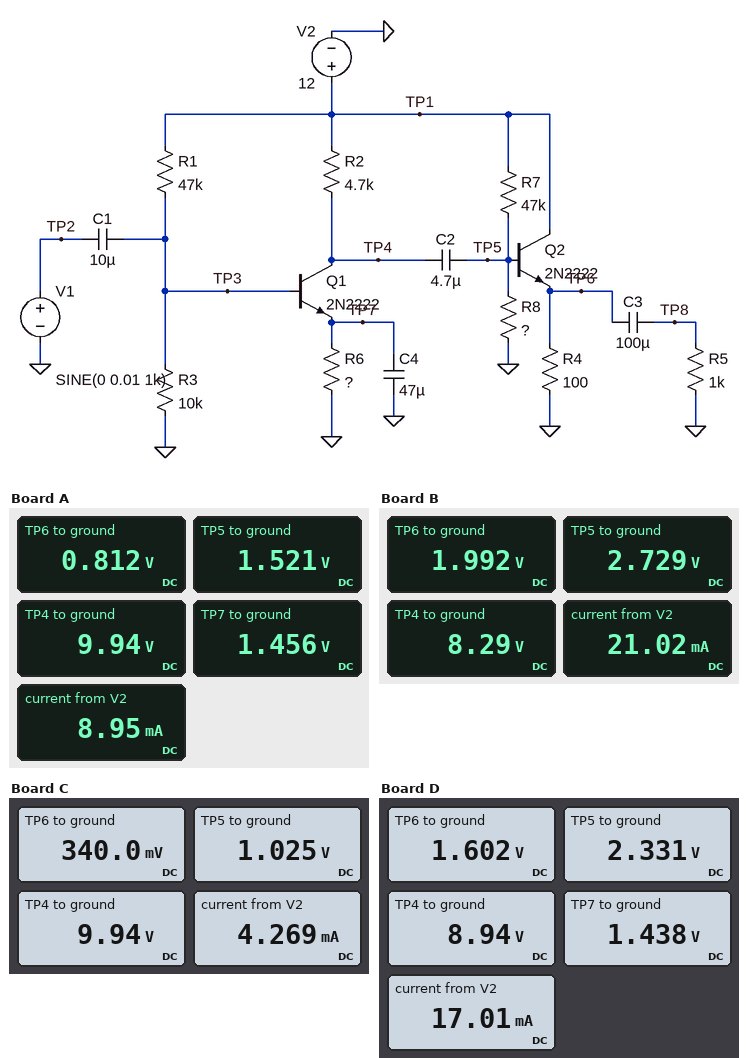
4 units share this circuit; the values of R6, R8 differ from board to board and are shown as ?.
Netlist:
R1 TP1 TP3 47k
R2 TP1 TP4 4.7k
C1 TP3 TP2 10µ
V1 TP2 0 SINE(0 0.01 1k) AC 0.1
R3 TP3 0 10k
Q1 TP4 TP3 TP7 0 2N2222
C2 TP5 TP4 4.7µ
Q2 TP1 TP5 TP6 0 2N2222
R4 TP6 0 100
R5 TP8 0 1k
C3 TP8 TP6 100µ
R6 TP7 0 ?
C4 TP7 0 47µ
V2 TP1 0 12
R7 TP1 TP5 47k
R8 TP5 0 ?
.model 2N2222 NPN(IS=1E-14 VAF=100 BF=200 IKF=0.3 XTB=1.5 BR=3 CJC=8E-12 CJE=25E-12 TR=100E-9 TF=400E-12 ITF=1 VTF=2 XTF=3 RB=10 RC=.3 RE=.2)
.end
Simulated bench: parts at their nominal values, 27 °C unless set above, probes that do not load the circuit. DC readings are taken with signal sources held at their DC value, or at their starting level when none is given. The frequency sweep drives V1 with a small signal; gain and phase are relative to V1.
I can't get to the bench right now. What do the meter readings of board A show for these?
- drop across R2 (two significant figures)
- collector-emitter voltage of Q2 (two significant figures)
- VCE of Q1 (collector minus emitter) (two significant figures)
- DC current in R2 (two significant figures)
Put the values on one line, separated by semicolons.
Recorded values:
2.1 V; 11 V; 8.5 V; 440 µA
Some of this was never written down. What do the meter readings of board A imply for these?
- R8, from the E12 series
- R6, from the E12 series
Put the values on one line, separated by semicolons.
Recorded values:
8.2 kΩ; 3.3 kΩ
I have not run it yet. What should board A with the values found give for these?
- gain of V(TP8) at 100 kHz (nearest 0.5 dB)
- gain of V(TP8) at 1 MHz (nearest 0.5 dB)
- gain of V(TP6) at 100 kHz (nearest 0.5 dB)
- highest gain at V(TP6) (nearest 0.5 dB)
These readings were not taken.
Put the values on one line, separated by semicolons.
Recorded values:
32.0 dB; 32.0 dB; 32.0 dB; 32.0 dB
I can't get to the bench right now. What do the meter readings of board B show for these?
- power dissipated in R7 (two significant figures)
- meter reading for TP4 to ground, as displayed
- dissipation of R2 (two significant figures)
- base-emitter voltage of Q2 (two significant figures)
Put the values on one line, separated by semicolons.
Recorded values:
1.8 mW; 8.29 V; 2.9 mW; 740 mV
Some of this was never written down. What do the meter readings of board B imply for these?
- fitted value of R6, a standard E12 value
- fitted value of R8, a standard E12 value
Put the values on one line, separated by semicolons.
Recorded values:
1.8 kΩ; 27 kΩ
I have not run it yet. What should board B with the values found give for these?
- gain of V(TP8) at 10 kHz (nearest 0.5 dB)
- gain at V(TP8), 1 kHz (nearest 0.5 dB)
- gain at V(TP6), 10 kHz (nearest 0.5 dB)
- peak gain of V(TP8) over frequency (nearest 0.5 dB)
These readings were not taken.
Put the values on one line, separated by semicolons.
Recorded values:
39.0 dB; 39.0 dB; 39.0 dB; 39.0 dB
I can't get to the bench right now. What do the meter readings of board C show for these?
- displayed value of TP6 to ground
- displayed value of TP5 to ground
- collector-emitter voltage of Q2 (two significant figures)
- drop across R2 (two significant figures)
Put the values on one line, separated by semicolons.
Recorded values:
340.0 mV; 1.025 V; 12 V; 2.1 V
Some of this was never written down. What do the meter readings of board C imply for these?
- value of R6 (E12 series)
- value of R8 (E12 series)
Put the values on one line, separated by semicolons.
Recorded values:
3.3 kΩ; 4.7 kΩ
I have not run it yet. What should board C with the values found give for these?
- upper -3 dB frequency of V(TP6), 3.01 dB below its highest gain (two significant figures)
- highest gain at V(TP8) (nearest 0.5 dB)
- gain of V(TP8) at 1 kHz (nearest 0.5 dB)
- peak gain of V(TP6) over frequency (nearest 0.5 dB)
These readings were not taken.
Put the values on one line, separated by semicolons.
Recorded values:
5.4 MHz; 30.0 dB; 30.0 dB; 30.0 dB
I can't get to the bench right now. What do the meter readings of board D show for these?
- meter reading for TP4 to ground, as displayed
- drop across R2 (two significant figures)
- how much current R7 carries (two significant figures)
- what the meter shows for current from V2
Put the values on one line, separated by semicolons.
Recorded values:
8.94 V; 3.1 V; 210 µA; 17.01 mA
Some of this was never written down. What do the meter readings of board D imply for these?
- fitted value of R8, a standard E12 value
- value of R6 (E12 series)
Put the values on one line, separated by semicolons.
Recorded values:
18 kΩ; 2.2 kΩ
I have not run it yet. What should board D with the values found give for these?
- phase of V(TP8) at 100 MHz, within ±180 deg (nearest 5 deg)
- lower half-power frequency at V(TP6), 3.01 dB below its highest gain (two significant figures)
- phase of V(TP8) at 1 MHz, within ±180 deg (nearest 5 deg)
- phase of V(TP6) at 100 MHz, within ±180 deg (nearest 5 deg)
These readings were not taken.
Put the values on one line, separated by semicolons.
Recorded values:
75 deg; 87 Hz; 165 deg; 75 deg
